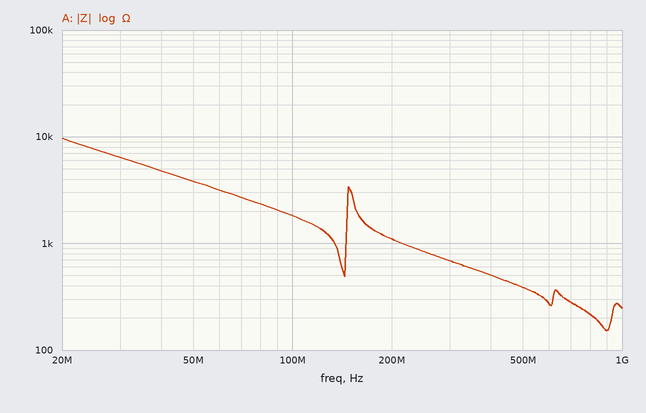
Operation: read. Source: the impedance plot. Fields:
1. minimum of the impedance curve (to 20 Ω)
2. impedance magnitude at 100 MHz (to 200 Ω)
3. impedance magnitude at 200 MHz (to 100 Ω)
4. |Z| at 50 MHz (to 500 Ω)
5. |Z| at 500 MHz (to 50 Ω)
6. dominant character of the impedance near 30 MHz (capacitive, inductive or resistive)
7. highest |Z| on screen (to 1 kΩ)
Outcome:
160 Ω
1.8 kΩ
1.1 kΩ
4.0 kΩ
400 Ω
capacitive
10 kΩ
